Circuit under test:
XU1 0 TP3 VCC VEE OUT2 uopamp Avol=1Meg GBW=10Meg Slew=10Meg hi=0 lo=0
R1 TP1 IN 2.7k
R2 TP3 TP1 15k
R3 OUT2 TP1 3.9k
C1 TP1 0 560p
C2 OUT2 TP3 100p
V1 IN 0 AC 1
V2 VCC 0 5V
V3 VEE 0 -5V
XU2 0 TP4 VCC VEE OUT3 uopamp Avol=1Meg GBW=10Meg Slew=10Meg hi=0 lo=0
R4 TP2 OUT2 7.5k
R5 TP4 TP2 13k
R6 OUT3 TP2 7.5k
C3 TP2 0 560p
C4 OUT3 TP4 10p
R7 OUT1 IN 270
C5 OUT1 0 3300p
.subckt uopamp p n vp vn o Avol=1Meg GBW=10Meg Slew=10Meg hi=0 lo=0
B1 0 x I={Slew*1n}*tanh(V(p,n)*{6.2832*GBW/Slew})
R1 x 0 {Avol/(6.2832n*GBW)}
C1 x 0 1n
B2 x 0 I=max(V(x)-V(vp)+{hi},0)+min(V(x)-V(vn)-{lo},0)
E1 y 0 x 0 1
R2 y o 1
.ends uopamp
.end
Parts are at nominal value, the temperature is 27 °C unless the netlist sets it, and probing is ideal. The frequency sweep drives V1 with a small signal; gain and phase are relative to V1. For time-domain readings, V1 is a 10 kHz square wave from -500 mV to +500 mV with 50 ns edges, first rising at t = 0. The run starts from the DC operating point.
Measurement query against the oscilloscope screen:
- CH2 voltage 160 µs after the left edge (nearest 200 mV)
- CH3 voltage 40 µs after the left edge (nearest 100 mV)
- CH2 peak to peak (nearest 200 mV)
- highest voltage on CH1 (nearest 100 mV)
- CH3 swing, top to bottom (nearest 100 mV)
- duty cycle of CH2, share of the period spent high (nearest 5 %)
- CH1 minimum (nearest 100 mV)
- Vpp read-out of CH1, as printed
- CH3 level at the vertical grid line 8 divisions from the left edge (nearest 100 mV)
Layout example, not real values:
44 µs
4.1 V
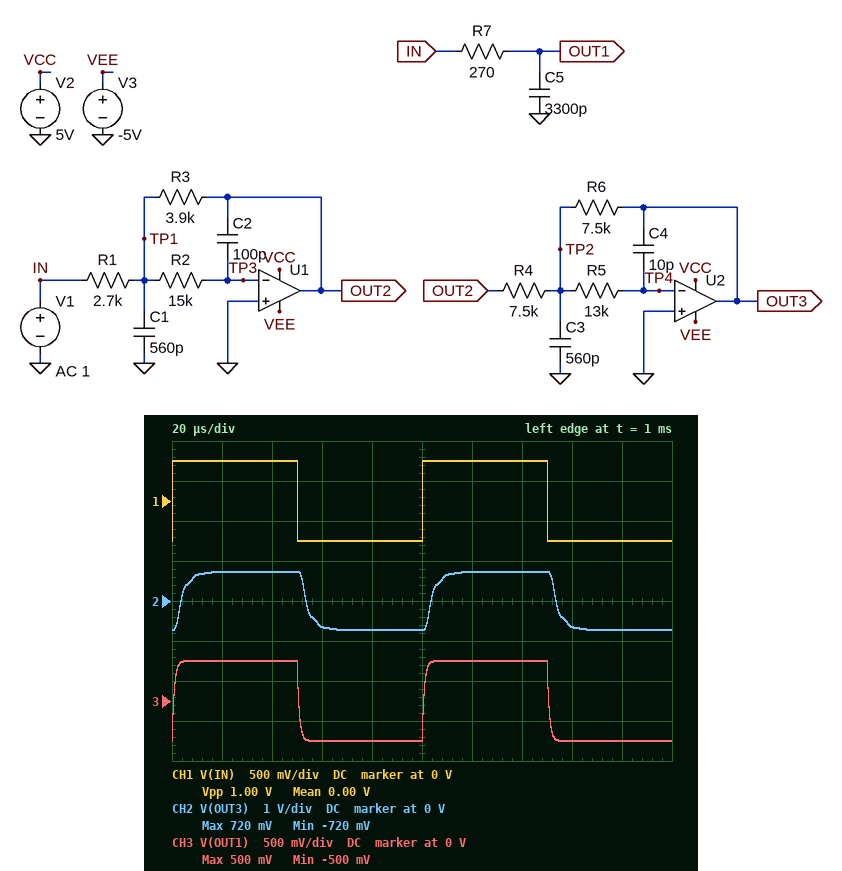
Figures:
-600 mV
500 mV
1.4 V
500 mV
1.0 V
50 %
-500 mV
1.00 V
-500 mV
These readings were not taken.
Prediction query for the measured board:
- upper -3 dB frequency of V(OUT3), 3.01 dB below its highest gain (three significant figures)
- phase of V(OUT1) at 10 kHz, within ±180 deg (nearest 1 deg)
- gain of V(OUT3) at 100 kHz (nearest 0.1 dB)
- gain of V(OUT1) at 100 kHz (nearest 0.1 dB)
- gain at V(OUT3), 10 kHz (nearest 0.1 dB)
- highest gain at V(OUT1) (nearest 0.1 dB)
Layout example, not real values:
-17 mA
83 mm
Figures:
53.5 kHz
-3 deg
-3.0 dB
-1.2 dB
3.0 dB
0 dB
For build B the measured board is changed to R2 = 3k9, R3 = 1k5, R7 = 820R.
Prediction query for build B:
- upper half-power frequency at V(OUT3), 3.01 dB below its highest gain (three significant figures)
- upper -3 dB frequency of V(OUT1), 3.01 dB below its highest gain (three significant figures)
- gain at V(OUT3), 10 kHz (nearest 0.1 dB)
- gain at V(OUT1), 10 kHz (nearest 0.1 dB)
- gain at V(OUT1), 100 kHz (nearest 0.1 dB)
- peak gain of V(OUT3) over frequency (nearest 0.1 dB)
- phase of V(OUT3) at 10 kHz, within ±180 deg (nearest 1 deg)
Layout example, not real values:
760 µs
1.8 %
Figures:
229 kHz
58.8 kHz
-5.1 dB
-0.1 dB
-5.9 dB
1.6 dB
-4 deg
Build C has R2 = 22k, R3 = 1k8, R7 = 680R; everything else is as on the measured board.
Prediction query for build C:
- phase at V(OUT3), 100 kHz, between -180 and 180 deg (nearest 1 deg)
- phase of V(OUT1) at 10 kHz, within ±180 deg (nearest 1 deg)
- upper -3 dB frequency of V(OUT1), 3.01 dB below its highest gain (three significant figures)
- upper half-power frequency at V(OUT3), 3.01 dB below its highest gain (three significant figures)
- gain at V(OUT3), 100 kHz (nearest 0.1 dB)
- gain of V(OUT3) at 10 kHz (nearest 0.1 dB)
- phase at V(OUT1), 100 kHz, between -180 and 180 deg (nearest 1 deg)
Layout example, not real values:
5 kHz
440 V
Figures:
-105 deg
-8 deg
70.9 kHz
54.3 kHz
-9.2 dB
-3.7 dB
-55 deg
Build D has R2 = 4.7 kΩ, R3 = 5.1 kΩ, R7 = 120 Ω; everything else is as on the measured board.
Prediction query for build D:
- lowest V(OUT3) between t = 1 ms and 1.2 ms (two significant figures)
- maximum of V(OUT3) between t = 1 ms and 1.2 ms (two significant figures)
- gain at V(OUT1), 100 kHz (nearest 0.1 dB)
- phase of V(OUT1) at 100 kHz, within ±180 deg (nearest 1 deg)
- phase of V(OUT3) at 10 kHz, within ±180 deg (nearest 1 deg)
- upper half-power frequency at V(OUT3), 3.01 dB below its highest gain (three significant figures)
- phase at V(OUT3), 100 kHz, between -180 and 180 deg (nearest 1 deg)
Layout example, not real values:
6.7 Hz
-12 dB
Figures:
-1.2 V
1.2 V
-0.3 dB
-14 deg
-8 deg
212 kHz
-87 deg
